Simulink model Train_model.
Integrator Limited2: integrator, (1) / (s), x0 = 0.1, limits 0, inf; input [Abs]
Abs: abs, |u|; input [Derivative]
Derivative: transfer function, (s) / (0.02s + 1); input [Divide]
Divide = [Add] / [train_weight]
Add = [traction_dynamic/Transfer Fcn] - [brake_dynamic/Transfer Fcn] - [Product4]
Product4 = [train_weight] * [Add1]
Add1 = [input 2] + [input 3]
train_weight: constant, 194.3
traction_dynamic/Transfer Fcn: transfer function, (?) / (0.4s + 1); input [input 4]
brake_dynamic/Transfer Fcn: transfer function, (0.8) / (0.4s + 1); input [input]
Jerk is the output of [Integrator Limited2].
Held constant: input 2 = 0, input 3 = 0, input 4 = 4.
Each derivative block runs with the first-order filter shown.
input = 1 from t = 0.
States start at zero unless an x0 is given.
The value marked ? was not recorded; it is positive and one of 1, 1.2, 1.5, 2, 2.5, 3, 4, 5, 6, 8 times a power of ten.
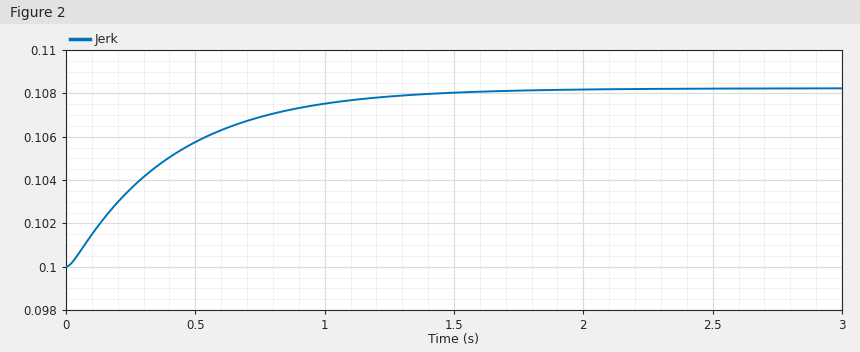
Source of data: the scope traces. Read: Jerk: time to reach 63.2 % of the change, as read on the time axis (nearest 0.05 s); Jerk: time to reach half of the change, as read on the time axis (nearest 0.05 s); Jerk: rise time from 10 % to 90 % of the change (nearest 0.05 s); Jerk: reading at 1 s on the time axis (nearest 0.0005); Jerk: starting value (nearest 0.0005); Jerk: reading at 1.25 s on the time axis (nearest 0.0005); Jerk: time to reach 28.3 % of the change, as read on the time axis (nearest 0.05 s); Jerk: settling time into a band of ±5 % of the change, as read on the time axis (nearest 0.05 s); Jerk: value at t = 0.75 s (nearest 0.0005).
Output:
0.40 s
0.30 s
0.90 s
0.1075
0.1000
0.1080
0.15 s
1.20 s
0.1070
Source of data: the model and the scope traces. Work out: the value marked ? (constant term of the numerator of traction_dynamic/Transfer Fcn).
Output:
0.6
